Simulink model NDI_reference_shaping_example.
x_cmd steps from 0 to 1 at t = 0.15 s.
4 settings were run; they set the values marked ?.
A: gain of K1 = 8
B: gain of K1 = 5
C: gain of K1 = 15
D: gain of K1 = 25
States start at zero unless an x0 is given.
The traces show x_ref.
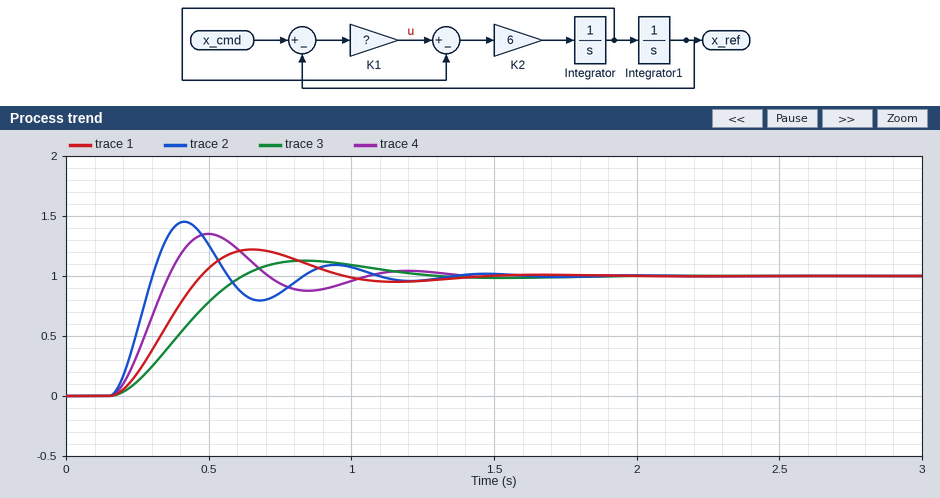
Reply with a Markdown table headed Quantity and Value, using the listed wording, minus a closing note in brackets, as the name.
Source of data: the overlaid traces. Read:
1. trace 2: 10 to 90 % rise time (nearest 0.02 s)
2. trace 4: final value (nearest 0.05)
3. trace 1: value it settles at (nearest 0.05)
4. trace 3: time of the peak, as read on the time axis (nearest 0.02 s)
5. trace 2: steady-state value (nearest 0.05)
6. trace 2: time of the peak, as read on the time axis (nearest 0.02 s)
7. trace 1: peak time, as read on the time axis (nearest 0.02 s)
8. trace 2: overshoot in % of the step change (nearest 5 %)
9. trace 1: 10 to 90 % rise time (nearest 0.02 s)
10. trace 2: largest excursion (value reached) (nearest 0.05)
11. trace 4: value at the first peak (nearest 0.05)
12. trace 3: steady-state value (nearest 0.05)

| Quantity | Value |
|---|---|
| trace 2: 10 to 90 % rise time | 0.10 s |
| trace 4: final value | 1.00 |
| trace 1: value it settles at | 1.00 |
| trace 3: time of the peak, as read on the time axis | 0.84 s |
| trace 2: steady-state value | 1.00 |
| trace 2: time of the peak, as read on the time axis | 0.42 s |
| trace 1: peak time, as read on the time axis | 0.66 s |
| trace 2: overshoot in % of the step change | 45 % |
| trace 1: 10 to 90 % rise time | 0.22 s |
| trace 2: largest excursion (value reached) | 1.45 |
| trace 4: value at the first peak | 1.35 |
| trace 3: steady-state value | 1.00 |
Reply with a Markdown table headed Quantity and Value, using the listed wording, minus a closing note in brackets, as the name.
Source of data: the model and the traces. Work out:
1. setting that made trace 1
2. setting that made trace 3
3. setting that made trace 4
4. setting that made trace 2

| Quantity | Value |
|---|---|
| setting that made trace 1 | A |
| setting that made trace 3 | B |
| setting that made trace 4 | C |
| setting that made trace 2 | D |
